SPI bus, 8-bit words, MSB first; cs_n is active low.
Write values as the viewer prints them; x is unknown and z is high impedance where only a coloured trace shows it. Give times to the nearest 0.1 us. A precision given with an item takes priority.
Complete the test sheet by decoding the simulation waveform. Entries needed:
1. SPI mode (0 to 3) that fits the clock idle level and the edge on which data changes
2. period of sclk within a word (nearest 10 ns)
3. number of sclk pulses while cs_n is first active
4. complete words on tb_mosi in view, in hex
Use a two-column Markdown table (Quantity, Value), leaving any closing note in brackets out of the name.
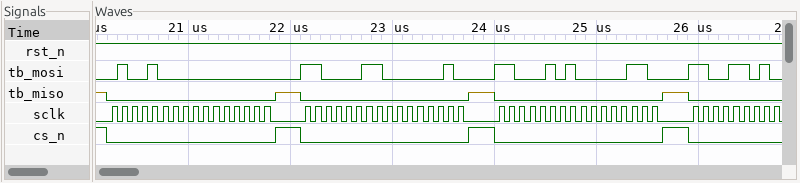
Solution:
| Quantity | Value |
|---|---|
| SPI mode (0 to 3) that fits the clock idle level and the edge on which data changes | 0 |
| period of sclk within a word | 100 ns |
| number of sclk pulses while cs_n is first active | 16 |
| complete words on tb_mosi in view, in hex | 48, 00, C3, 02, C5, 06, CD |
